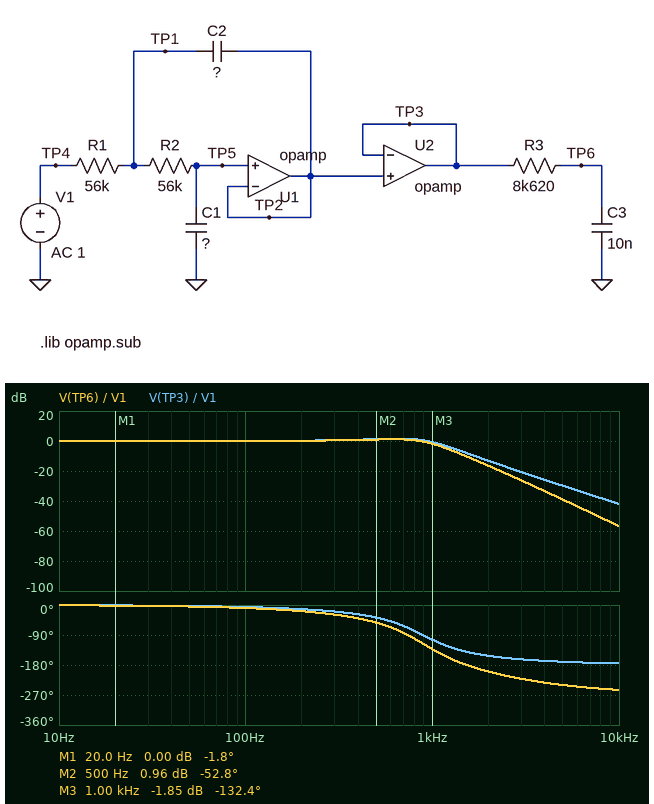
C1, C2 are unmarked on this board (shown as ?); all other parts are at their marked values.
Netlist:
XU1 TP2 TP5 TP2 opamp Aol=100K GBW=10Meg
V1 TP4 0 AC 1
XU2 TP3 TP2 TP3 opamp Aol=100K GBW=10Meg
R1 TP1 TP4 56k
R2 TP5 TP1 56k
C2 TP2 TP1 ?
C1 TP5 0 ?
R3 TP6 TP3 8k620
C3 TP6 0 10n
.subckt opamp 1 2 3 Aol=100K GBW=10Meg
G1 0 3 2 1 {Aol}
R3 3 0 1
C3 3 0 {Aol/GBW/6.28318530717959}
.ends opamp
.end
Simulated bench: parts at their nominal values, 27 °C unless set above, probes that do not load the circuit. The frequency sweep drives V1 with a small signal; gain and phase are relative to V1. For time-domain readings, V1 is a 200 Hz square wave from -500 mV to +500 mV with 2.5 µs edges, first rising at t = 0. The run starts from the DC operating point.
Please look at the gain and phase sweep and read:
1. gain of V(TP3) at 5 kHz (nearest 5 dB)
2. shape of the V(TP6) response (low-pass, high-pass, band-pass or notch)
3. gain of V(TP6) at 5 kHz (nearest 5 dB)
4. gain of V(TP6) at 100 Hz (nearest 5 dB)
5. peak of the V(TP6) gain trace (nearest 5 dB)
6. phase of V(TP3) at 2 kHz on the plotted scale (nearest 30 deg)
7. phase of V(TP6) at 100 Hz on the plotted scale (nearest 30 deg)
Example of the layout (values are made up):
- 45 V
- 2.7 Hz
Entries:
- -30 dB
- low-pass
- -40 dB
- 0 dB
- 0 dB
- -150 deg
- 0 deg
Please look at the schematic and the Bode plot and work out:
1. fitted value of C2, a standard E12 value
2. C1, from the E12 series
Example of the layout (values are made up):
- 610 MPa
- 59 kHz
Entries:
- 6.8 nF
- 1.5 nF
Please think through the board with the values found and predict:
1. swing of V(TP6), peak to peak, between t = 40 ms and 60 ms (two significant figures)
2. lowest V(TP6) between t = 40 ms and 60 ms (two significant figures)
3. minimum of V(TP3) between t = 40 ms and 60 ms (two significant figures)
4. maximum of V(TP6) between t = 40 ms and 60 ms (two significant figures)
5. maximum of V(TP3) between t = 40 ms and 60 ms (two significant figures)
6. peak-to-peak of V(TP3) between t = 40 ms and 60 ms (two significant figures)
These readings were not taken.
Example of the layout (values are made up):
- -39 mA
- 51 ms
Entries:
- 1.3 V
- -660 mV
- -690 mV
- 660 mV
- 690 mV
- 1.4 V
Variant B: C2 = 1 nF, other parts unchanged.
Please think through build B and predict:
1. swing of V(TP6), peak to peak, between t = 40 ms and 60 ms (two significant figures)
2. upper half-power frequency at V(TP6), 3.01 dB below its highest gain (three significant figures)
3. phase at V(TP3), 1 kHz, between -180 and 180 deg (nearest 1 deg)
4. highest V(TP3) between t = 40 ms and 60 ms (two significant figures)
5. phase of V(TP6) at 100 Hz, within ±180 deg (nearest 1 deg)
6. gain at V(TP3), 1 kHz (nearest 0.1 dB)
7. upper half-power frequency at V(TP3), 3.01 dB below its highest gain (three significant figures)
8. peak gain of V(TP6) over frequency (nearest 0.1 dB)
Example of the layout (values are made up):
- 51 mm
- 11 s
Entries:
- 1.0 V
- 896 Hz
- -52 deg
- 500 mV
- -9 deg
- -2.5 dB
- 1.13 kHz
- 0 dB
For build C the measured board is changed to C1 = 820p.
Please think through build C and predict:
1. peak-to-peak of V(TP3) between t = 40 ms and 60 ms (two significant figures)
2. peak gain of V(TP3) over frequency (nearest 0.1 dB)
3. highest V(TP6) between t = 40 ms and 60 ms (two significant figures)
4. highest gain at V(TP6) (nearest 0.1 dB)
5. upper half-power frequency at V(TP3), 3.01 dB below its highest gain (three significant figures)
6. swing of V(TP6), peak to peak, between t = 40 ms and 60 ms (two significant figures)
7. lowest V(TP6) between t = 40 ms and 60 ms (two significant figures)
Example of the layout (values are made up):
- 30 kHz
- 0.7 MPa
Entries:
- 1.6 V
- 3.7 dB
- 750 mV
- 2.6 dB
- 1.43 kHz
- 1.5 V
- -750 mV
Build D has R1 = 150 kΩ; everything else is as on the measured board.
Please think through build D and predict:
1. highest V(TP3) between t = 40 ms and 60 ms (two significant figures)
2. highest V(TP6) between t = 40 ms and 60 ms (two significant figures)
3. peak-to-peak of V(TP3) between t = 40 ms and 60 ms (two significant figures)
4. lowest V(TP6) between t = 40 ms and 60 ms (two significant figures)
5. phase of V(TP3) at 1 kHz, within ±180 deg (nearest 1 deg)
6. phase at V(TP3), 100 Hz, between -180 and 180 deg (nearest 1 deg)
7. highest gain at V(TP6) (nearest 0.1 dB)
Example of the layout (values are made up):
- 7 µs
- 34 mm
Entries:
- 640 mV
- 630 mV
- 1.3 V
- -630 mV
- -141 deg
- -11 deg
- 0.8 dB
